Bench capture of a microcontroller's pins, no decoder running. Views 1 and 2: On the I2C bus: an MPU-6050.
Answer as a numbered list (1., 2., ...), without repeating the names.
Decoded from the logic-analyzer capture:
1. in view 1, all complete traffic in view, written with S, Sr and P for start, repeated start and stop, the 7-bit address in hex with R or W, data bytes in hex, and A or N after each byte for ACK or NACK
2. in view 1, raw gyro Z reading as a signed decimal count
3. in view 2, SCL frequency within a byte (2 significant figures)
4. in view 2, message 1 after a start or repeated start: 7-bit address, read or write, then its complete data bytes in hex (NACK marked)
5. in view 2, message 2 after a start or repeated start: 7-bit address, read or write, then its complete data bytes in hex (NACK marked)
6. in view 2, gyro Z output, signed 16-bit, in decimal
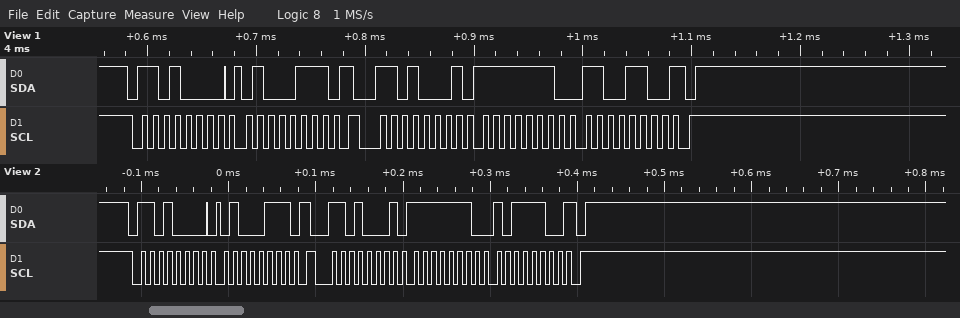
1. S 68W A 47 A Sr 68R A FE A CC N P
2. -308
3. 100 kHz
4. 0x68 write: 47
5. 0x68 read: FE BC NACK
6. -324
